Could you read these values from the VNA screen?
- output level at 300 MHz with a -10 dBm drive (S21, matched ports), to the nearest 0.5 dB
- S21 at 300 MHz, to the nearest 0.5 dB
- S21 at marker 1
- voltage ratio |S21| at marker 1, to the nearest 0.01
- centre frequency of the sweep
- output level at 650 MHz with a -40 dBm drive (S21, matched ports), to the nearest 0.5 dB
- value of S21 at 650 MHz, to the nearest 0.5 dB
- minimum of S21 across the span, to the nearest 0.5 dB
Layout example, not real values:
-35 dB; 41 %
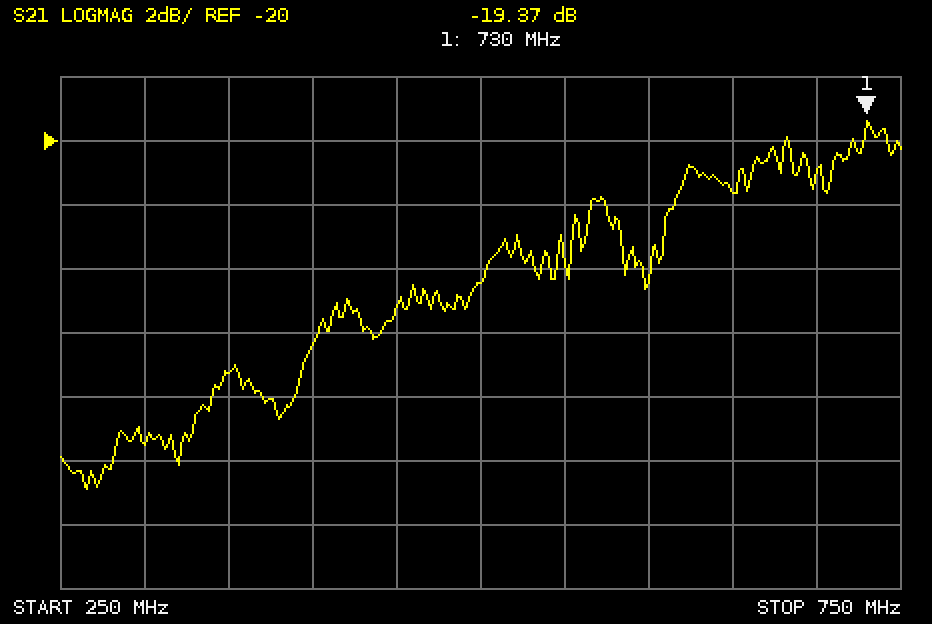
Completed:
-39.5 dBm; -29.5 dB; -19.37 dB; 0.11; 500 MHz; -61.5 dBm; -21.5 dB; -31.0 dB
